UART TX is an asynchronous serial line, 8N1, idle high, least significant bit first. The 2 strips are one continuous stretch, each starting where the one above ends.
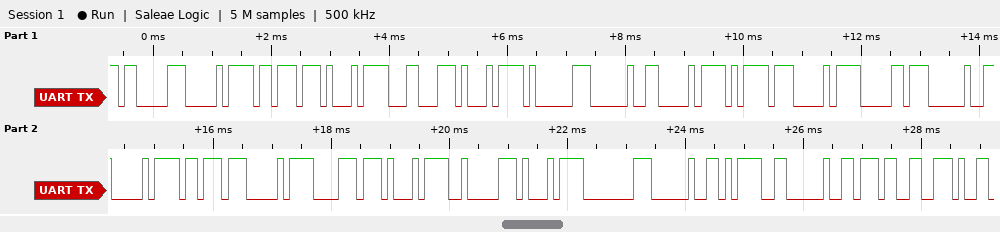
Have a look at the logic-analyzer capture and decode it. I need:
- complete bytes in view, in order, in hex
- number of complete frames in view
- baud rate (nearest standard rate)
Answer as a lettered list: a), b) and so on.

a) 83 D0 BB D1 8C D1 81 20 D0 BD D0 B0 20 D0 BB D0 B8 D1 82 D1 80 20 3D 20 37 2E
b) 26
c) 9600 baud
